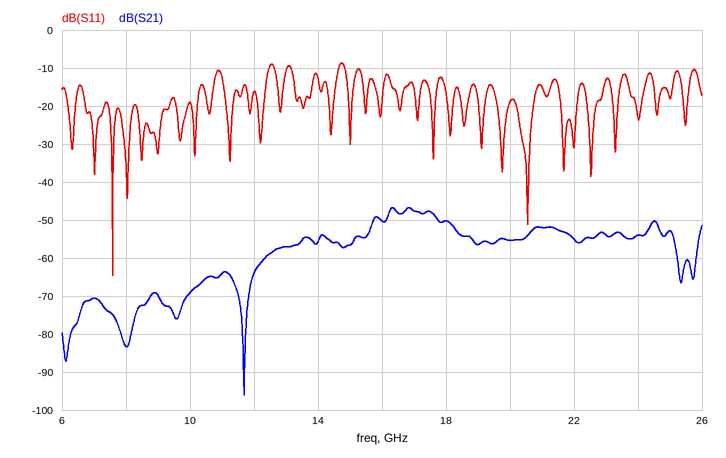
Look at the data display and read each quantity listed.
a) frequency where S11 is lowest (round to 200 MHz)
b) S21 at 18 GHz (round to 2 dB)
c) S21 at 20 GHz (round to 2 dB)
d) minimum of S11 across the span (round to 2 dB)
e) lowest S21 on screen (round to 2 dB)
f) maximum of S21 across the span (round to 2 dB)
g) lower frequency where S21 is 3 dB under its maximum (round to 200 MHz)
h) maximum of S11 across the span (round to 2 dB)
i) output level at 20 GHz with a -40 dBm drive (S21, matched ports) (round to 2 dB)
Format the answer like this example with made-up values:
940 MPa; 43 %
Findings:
7.6 GHz; -50 dB; -56 dB; -64 dB; -96 dB; -46 dB; 16.2 GHz; -8 dB; -96 dBm
